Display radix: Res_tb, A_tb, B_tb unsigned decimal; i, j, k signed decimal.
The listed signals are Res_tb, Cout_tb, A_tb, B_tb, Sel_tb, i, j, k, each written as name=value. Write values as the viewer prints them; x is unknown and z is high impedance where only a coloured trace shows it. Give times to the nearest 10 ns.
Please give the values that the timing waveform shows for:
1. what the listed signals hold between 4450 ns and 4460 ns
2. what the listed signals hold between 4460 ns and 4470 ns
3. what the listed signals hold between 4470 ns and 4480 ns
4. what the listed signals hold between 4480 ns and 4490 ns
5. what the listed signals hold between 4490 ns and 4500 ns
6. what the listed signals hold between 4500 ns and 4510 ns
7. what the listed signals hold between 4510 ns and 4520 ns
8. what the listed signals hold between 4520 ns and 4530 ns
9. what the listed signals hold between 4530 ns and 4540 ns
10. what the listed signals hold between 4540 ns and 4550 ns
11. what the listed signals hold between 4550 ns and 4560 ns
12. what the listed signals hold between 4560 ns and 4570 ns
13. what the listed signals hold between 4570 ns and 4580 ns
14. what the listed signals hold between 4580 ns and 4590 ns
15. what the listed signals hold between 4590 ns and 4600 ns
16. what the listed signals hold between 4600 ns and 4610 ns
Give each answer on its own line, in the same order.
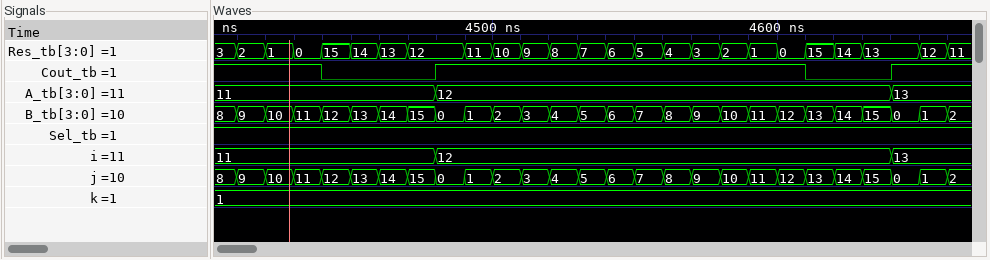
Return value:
Res_tb=14, Cout_tb=0, A_tb=11, B_tb=13, Sel_tb=1, i=11, j=13, k=1
Res_tb=13, Cout_tb=0, A_tb=11, B_tb=14, Sel_tb=1, i=11, j=14, k=1
Res_tb=12, Cout_tb=0, A_tb=11, B_tb=15, Sel_tb=1, i=11, j=15, k=1
Res_tb=12, Cout_tb=1, A_tb=12, B_tb=0, Sel_tb=1, i=12, j=0, k=1
Res_tb=11, Cout_tb=1, A_tb=12, B_tb=1, Sel_tb=1, i=12, j=1, k=1
Res_tb=10, Cout_tb=1, A_tb=12, B_tb=2, Sel_tb=1, i=12, j=2, k=1
Res_tb=9, Cout_tb=1, A_tb=12, B_tb=3, Sel_tb=1, i=12, j=3, k=1
Res_tb=8, Cout_tb=1, A_tb=12, B_tb=4, Sel_tb=1, i=12, j=4, k=1
Res_tb=7, Cout_tb=1, A_tb=12, B_tb=5, Sel_tb=1, i=12, j=5, k=1
Res_tb=6, Cout_tb=1, A_tb=12, B_tb=6, Sel_tb=1, i=12, j=6, k=1
Res_tb=5, Cout_tb=1, A_tb=12, B_tb=7, Sel_tb=1, i=12, j=7, k=1
Res_tb=4, Cout_tb=1, A_tb=12, B_tb=8, Sel_tb=1, i=12, j=8, k=1
Res_tb=3, Cout_tb=1, A_tb=12, B_tb=9, Sel_tb=1, i=12, j=9, k=1
Res_tb=2, Cout_tb=1, A_tb=12, B_tb=10, Sel_tb=1, i=12, j=10, k=1
Res_tb=1, Cout_tb=1, A_tb=12, B_tb=11, Sel_tb=1, i=12, j=11, k=1
Res_tb=0, Cout_tb=1, A_tb=12, B_tb=12, Sel_tb=1, i=12, j=12, k=1
